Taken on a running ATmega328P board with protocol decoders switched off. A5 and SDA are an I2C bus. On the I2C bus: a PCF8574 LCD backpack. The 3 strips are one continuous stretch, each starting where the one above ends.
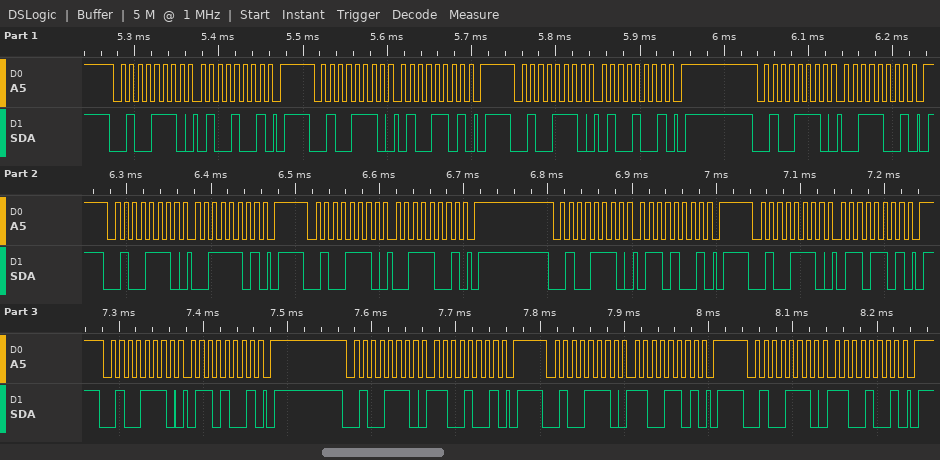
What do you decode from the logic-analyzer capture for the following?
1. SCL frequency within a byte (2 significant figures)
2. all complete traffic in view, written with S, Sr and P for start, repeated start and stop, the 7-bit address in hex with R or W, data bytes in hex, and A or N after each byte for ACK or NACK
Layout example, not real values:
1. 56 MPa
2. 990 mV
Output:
1. 100 kHz
2. S 27W A 49 A P S 27W A 4D A P S 27W A 49 A P S 27W A 39 A P S 27W A 3D A P S 27W A 39 A P S 27W A 69 A P S 27W A 6D A P S 27W A 69 A P S 27W A C9 A P S 27W A CD A P S 27W A C9 A P
